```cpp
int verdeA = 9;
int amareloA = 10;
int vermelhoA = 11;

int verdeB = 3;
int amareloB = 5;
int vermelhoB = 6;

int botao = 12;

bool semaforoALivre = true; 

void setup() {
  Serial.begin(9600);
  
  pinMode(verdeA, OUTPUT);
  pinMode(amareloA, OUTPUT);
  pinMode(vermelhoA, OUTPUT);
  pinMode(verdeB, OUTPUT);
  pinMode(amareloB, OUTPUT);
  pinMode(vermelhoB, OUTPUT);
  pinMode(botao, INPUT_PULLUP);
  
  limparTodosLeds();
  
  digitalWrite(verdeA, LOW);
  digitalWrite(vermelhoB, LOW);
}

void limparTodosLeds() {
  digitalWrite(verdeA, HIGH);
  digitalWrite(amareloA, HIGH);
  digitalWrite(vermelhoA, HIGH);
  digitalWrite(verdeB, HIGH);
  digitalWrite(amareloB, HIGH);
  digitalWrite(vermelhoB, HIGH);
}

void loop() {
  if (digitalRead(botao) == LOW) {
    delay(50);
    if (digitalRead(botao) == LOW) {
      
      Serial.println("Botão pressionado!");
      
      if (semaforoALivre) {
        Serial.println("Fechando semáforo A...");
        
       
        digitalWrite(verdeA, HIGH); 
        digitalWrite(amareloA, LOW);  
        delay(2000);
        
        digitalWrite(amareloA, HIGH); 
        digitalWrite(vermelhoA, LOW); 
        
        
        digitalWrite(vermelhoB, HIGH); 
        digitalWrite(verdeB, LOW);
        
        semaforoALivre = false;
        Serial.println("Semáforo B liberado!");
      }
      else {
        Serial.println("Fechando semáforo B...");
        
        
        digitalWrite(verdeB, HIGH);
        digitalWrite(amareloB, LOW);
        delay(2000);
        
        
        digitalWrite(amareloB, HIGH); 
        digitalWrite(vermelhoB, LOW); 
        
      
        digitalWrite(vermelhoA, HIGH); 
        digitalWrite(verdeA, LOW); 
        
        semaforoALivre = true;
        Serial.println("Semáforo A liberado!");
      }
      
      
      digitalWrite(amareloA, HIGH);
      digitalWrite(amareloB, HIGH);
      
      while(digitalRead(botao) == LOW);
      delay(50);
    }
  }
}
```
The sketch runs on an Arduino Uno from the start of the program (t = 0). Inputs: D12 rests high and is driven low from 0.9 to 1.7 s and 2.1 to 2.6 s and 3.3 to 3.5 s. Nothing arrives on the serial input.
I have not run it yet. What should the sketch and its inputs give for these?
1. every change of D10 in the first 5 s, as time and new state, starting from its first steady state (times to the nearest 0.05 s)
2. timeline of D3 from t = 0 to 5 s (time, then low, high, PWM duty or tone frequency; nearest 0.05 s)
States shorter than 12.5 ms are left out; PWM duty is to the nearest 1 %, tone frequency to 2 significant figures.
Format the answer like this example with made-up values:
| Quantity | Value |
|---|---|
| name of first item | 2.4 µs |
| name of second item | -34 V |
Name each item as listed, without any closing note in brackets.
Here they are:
| Quantity | Value |
|---|---|
| every change of D10 in the first 5 s, as time and new state, starting from its first steady state | 0 s high; 0.95 s low; 2.95 s high |
| timeline of D3 from t = 0 to 5 s | 0 s high; 2.95 s low; 3.35 s high |
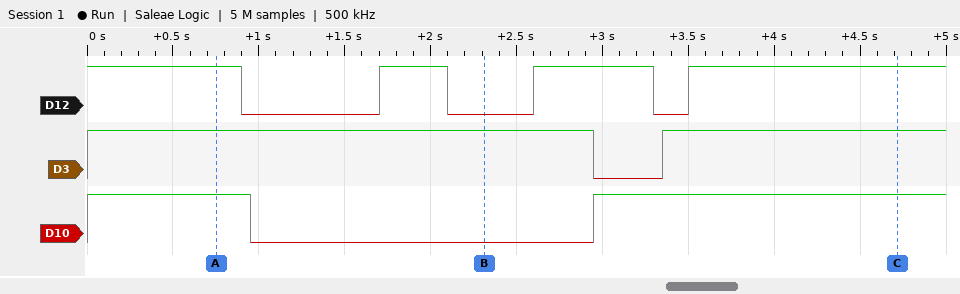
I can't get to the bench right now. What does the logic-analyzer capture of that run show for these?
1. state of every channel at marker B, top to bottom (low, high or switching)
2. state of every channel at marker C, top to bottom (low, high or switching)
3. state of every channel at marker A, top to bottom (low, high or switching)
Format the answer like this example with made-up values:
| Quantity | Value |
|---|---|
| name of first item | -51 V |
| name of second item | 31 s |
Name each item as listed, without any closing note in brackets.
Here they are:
| Quantity | Value |
|---|---|
| state of every channel at marker B, top to bottom | D12 low, D3 high, D10 low |
| state of every channel at marker C, top to bottom | D12 high, D3 high, D10 high |
| state of every channel at marker A, top to bottom | D12 high, D3 high, D10 high |
